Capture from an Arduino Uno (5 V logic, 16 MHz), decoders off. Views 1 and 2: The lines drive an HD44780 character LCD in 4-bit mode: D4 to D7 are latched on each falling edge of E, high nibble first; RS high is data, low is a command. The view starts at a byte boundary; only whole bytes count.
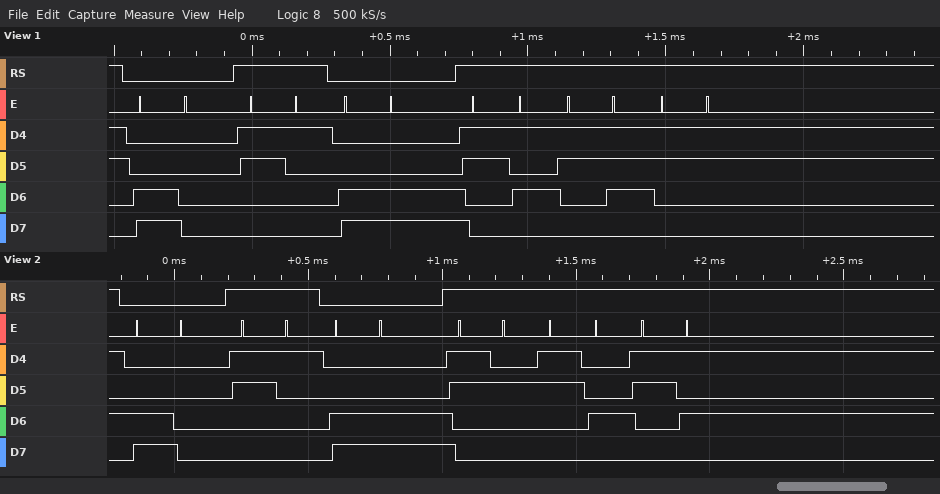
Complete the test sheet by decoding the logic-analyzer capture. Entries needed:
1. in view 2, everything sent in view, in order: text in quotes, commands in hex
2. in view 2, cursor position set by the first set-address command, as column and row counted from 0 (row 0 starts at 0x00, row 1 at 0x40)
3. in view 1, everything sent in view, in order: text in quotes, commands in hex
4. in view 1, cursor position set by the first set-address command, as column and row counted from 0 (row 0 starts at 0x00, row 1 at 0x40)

0xC0 "1" 0xCC "245"
column 0, row 1
0xC0 "1" 0xCC "573"
column 0, row 1
